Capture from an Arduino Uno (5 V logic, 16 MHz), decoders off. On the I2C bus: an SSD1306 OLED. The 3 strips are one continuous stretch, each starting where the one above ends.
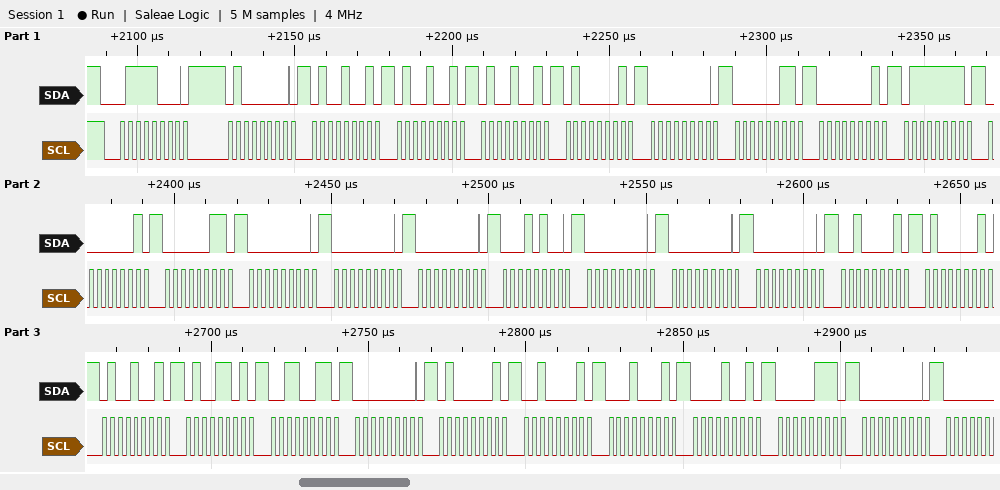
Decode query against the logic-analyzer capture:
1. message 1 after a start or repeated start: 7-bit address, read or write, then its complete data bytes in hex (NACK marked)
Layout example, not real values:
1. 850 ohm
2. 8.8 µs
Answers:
1. 0x3C write: 40 49 49 49 41 00 03 01 7F 01 03 00 00 00 14 00 00 00 21 41 49 4D 33 00 41 21 11 09 07 00
